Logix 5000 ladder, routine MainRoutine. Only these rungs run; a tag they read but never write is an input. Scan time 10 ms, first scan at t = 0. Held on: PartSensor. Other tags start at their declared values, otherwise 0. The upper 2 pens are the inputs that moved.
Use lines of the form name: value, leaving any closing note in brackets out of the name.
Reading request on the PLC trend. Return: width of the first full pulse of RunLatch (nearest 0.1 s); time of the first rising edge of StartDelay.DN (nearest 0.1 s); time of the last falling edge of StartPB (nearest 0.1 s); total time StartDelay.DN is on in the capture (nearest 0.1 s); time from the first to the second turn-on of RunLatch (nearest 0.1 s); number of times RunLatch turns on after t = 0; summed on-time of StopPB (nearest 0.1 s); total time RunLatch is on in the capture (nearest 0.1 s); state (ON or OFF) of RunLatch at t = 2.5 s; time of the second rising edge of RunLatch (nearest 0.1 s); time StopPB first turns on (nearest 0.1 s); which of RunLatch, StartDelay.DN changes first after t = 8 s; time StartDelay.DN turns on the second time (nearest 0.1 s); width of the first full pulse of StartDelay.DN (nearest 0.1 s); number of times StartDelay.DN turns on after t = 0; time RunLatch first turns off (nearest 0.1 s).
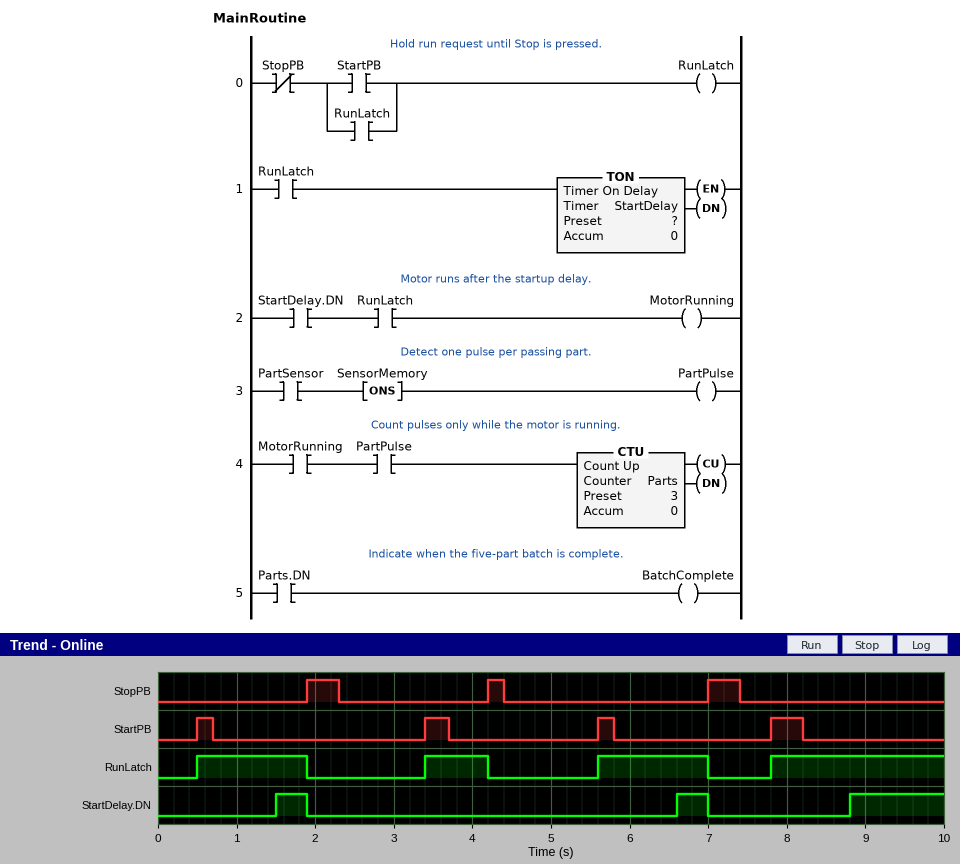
width of the first full pulse of RunLatch: 1.4 s
time of the first rising edge of StartDelay.DN: 1.5 s
time of the last falling edge of StartPB: 8.2 s
total time StartDelay.DN is on in the capture: 2.0 s
time from the first to the second turn-on of RunLatch: 2.9 s
number of times RunLatch turns on after t = 0: 4
summed on-time of StopPB: 1.0 s
total time RunLatch is on in the capture: 5.8 s
state (ON or OFF) of RunLatch at t = 2.5 s: OFF
time of the second rising edge of RunLatch: 3.4 s
time StopPB first turns on: 1.9 s
which of RunLatch, StartDelay.DN changes first after t = 8 s: StartDelay.DN
time StartDelay.DN turns on the second time: 6.6 s
width of the first full pulse of StartDelay.DN: 0.4 s
number of times StartDelay.DN turns on after t = 0: 3
time RunLatch first turns off: 1.9 s
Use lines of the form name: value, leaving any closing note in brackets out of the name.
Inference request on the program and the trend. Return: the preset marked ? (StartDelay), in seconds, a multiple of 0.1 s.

the preset marked ? (StartDelay), in seconds, a multiple of 0.1 s: 1.0 s
